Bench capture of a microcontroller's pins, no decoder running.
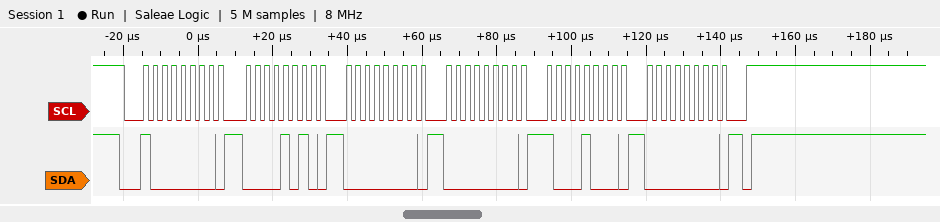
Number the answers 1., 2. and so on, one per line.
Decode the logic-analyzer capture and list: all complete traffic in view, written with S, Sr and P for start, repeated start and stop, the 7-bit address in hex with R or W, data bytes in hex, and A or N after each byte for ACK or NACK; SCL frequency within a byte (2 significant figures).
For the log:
1. S 40W A 0A A 00 A 00 A 88 A 00 A P
2. 400 kHz
